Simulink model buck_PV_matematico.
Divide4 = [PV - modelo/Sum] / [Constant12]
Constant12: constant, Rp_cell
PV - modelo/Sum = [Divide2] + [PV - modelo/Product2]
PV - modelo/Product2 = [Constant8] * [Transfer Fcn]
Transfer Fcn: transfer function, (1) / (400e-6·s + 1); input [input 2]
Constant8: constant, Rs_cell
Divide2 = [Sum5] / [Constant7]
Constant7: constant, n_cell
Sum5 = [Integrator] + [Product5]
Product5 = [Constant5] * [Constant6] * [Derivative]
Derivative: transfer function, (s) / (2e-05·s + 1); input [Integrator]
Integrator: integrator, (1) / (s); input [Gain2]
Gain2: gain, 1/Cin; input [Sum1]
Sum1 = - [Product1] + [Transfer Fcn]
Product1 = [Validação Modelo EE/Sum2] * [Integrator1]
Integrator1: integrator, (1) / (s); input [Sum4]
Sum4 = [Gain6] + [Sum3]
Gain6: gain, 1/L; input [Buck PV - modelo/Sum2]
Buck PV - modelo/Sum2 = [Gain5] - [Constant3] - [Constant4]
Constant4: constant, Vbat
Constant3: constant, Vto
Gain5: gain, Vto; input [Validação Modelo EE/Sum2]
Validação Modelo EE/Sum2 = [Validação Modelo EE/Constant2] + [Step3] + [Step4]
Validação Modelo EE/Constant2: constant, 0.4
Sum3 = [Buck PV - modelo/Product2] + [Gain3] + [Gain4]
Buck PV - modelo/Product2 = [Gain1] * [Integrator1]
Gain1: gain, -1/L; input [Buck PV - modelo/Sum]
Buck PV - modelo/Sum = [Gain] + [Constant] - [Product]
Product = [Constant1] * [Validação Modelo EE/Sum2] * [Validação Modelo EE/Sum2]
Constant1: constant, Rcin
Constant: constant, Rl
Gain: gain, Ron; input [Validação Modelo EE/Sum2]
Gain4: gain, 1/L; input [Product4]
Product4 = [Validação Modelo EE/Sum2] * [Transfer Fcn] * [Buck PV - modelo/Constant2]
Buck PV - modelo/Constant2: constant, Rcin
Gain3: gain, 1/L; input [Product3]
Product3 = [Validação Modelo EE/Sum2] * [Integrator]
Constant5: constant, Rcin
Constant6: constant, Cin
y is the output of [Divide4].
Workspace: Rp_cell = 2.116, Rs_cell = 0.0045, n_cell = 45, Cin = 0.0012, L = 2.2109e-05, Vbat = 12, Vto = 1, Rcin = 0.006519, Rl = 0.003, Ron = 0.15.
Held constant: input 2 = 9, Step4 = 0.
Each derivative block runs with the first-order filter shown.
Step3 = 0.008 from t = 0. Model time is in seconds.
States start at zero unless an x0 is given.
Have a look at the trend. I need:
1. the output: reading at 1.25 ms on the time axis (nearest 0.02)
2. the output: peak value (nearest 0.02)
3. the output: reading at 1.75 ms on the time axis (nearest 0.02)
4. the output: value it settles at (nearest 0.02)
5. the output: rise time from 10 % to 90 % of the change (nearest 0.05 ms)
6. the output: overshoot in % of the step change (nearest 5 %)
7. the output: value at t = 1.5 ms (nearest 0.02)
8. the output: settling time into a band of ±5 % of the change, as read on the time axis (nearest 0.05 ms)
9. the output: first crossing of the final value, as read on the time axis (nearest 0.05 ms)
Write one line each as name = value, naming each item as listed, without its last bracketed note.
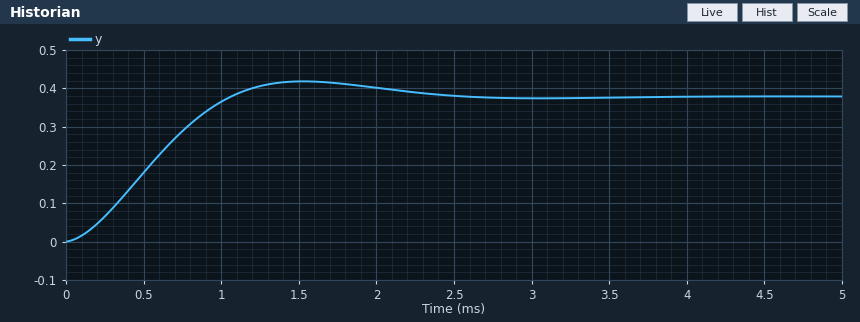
the output: reading at 1.25 ms on the time axis = 0.40
the output: peak value = 0.42
the output: reading at 1.75 ms on the time axis = 0.42
the output: value it settles at = 0.38
the output: rise time from 10 % to 90 % of the change = 0.75 ms
the output: overshoot in % of the step change = 10 %
the output: value at t = 1.5 ms = 0.42
the output: settling time into a band of ±5 % of the change, as read on the time axis = 2.10 ms
the output: first crossing of the final value, as read on the time axis = 1.05 ms
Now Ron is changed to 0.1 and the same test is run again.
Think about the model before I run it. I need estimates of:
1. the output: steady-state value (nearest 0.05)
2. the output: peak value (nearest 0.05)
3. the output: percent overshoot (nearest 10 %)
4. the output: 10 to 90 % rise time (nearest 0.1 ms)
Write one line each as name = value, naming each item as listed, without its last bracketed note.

the output: steady-state value = 0.35
the output: peak value = 0.45
the output: percent overshoot = 30 %
the output: 10 to 90 % rise time = 0.6 ms
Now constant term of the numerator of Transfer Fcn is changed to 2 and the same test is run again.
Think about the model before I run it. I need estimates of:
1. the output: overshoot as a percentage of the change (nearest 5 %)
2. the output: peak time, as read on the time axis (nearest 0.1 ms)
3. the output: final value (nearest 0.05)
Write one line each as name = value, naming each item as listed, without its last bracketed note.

the output: overshoot as a percentage of the change = 10 %
the output: peak time, as read on the time axis = 1.5 ms
the output: final value = 0.45
